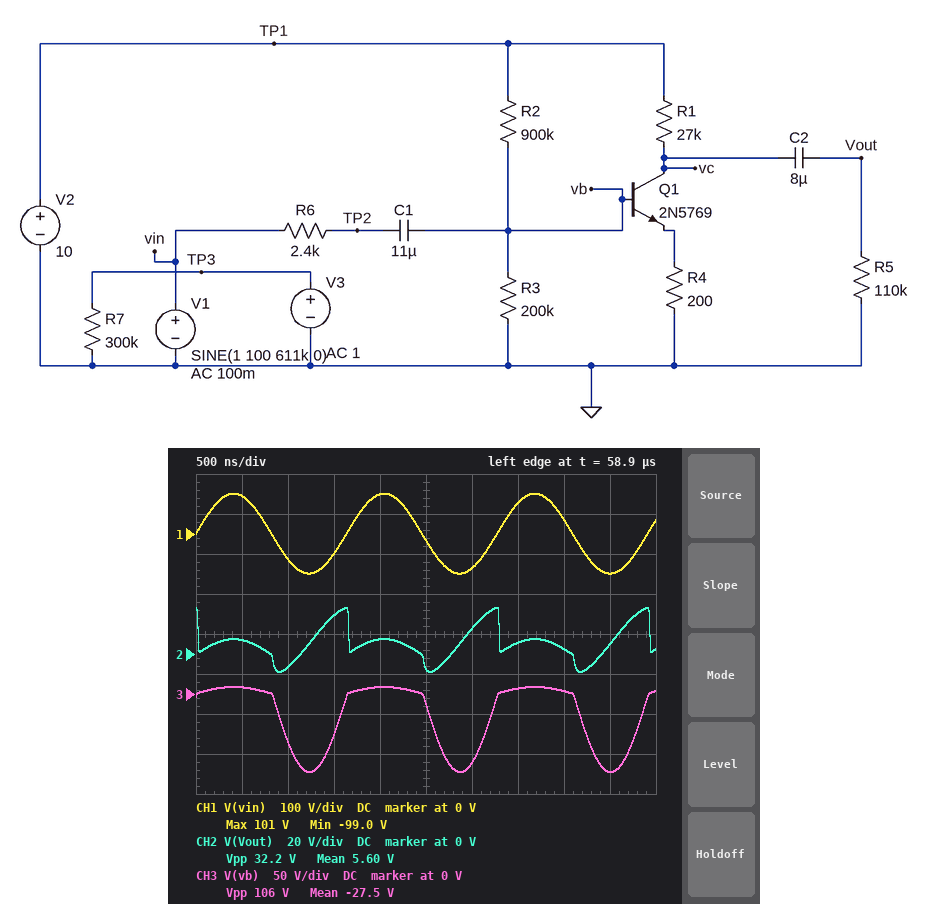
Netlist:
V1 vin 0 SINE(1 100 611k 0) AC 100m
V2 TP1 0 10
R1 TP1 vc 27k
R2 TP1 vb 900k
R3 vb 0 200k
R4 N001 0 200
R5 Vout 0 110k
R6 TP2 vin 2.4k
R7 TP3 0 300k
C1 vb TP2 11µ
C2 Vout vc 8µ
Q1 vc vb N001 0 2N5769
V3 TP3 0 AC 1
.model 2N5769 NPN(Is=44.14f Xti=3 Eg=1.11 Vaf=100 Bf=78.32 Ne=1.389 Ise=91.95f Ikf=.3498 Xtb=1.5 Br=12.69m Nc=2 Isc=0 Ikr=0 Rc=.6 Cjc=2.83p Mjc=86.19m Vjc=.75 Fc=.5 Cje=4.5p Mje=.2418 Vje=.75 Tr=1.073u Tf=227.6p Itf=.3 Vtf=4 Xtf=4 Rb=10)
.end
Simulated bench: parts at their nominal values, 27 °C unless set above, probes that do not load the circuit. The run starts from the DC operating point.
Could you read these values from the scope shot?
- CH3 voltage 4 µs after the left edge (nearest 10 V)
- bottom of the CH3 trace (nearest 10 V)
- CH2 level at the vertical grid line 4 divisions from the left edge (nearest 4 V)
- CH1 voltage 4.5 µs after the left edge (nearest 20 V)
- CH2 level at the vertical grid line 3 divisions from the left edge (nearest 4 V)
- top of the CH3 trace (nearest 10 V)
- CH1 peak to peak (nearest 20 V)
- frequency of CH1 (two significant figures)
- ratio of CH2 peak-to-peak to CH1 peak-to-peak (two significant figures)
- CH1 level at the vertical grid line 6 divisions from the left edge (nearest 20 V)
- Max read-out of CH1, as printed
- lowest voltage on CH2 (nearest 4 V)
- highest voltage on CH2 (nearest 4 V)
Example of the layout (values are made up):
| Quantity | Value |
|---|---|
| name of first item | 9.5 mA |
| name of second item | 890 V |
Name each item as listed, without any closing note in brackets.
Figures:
| Quantity | Value |
|---|---|
| CH3 voltage 4 µs after the left edge | 0 V |
| bottom of the CH3 trace | -100 V |
| CH2 level at the vertical grid line 4 divisions from the left edge | 8 V |
| CH1 voltage 4.5 µs after the left edge | -100 V |
| CH2 level at the vertical grid line 3 divisions from the left edge | 20 V |
| top of the CH3 trace | 10 V |
| CH1 peak to peak | 200 V |
| frequency of CH1 | 610 kHz |
| ratio of CH2 peak-to-peak to CH1 peak-to-peak | 0.16 |
| CH1 level at the vertical grid line 6 divisions from the left edge | -80 V |
| Max read-out of CH1, as printed | 101 V |
| lowest voltage on CH2 | -8 V |
| highest voltage on CH2 | 24 V |
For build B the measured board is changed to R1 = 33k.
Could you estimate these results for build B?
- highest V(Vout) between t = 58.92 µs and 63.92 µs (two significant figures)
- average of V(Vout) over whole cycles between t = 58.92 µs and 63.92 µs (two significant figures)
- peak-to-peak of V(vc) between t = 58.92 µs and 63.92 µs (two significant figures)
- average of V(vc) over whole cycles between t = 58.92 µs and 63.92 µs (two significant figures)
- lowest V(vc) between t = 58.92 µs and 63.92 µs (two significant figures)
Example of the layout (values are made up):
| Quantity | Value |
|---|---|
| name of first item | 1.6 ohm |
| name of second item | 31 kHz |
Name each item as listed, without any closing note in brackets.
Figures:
| Quantity | Value |
|---|---|
| highest V(Vout) between t = 58.92 µs and 63.92 µs | 25 V |
| average of V(Vout) over whole cycles between t = 58.92 µs and 63.92 µs | 5.3 V |
| peak-to-peak of V(vc) between t = 58.92 µs and 63.92 µs | 37 V |
| average of V(vc) over whole cycles between t = 58.92 µs and 63.92 µs | 5.6 V |
| lowest V(vc) between t = 58.92 µs and 63.92 µs | -11 V |
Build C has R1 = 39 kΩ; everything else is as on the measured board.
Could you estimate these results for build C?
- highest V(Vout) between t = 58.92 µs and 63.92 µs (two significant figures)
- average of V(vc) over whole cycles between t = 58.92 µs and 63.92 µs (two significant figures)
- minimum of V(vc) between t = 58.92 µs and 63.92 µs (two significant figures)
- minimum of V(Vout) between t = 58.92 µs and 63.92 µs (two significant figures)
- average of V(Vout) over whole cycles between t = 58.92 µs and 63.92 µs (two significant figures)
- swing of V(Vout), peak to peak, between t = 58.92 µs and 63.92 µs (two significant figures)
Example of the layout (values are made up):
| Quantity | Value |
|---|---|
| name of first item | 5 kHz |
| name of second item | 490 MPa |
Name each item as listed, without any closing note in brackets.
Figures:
| Quantity | Value |
|---|---|
| highest V(Vout) between t = 58.92 µs and 63.92 µs | 27 V |
| average of V(vc) over whole cycles between t = 58.92 µs and 63.92 µs | 5.2 V |
| minimum of V(vc) between t = 58.92 µs and 63.92 µs | -13 V |
| minimum of V(Vout) between t = 58.92 µs and 63.92 µs | -14 V |
| average of V(Vout) over whole cycles between t = 58.92 µs and 63.92 µs | 5.0 V |
| swing of V(Vout), peak to peak, between t = 58.92 µs and 63.92 µs | 41 V |
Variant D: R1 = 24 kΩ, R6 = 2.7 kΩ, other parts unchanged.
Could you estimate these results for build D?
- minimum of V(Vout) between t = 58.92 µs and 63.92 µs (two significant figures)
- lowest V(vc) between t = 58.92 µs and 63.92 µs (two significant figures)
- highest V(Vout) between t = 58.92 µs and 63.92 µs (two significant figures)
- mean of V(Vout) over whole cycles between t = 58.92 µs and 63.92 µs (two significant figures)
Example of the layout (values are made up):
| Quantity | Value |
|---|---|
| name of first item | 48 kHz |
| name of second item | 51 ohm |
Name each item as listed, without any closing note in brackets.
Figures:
| Quantity | Value |
|---|---|
| minimum of V(Vout) between t = 58.92 µs and 63.92 µs | -7.6 V |
| lowest V(vc) between t = 58.92 µs and 63.92 µs | -7.2 V |
| highest V(Vout) between t = 58.92 µs and 63.92 µs | 22 V |
| mean of V(Vout) over whole cycles between t = 58.92 µs and 63.92 µs | 5.5 V |
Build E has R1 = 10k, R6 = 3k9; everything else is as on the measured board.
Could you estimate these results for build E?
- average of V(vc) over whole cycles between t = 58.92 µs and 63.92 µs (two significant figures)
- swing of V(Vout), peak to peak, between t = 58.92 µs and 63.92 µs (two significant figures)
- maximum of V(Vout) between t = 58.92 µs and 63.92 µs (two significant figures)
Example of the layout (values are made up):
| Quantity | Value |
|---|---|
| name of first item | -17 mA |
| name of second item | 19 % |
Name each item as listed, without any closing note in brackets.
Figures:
| Quantity | Value |
|---|---|
| average of V(vc) over whole cycles between t = 58.92 µs and 63.92 µs | 6.4 V |
| swing of V(Vout), peak to peak, between t = 58.92 µs and 63.92 µs | 16 V |
| maximum of V(Vout) between t = 58.92 µs and 63.92 µs | 11 V |
